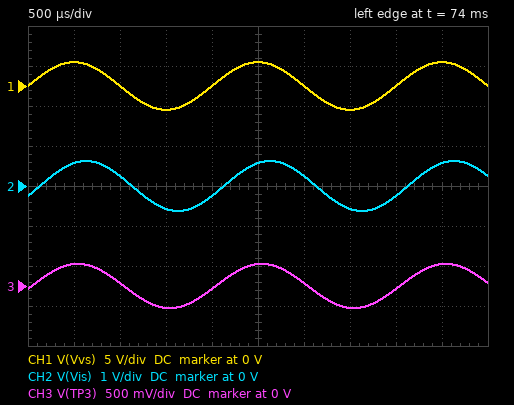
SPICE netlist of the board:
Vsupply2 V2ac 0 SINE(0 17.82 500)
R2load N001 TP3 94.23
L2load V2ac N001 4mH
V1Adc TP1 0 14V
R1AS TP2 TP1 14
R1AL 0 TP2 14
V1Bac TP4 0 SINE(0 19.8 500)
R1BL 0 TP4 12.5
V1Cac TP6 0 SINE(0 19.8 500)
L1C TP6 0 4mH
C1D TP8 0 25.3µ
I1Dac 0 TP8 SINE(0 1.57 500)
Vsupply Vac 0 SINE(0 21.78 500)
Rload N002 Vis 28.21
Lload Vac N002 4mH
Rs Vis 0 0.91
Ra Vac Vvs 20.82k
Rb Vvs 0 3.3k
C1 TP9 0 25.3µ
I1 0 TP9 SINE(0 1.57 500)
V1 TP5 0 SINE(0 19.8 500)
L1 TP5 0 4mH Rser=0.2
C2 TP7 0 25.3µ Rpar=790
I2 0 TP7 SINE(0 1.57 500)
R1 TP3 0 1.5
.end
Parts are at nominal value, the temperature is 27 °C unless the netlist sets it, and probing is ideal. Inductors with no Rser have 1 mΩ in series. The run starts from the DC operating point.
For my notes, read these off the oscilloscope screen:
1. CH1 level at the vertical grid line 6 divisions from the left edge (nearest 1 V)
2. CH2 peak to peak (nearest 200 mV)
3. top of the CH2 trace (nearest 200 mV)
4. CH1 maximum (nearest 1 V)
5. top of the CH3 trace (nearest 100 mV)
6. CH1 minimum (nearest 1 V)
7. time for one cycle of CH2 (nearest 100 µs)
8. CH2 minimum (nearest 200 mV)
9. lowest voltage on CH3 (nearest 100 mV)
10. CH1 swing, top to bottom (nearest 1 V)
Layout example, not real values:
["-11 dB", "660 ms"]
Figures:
["0 V", "1.2 V", "600 mV", "3 V", "300 mV", "-3 V", "2.0 ms", "-600 mV", "-300 mV", "6 V"]
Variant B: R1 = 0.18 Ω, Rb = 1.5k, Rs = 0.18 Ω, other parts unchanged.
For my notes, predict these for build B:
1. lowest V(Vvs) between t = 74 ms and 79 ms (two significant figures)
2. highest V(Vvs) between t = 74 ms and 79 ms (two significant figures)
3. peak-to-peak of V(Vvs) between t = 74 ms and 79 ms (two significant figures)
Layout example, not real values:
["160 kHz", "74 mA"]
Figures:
["-1.5 V", "1.5 V", "2.9 V"]
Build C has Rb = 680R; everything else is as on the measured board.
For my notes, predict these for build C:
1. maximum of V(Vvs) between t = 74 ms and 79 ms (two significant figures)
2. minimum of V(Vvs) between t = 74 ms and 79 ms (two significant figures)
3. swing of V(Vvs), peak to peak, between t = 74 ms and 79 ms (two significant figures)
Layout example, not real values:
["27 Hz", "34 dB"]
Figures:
["690 mV", "-690 mV", "1.4 V"]
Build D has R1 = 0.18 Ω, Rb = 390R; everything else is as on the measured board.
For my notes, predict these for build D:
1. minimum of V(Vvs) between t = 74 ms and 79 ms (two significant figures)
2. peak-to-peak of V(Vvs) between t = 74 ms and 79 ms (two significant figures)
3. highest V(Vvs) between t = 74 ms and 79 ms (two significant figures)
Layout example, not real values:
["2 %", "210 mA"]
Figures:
["-400 mV", "800 mV", "400 mV"]
